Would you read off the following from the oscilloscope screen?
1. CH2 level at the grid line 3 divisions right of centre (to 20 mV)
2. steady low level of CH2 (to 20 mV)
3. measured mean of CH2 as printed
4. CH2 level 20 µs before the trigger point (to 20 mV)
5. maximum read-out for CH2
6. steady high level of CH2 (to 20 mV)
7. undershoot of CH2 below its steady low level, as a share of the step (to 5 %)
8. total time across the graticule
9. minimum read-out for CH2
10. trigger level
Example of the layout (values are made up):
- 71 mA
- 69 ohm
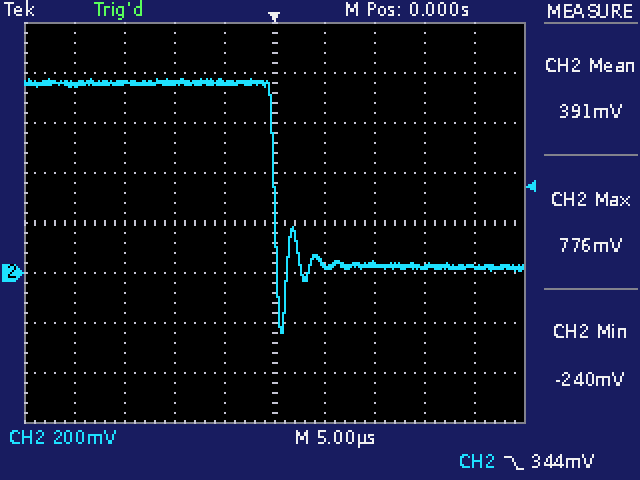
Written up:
- 20 mV
- 20 mV
- 391 mV
- 760 mV
- 776 mV
- 760 mV
- 35 %
- 50 µs
- -240 mV
- 344 mV
